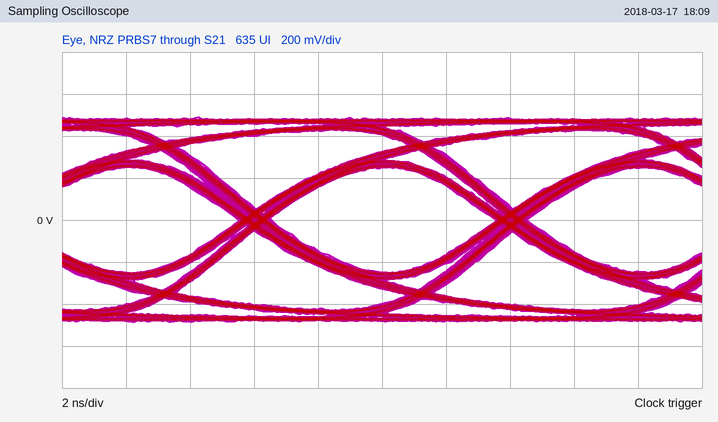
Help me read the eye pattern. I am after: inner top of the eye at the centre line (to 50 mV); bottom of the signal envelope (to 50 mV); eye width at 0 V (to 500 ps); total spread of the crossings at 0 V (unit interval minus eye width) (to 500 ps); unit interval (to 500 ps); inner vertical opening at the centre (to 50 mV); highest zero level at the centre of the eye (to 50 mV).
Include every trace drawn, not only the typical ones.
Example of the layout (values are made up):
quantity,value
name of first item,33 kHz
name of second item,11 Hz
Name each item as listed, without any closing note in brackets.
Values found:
quantity,value
inner top of the eye at the centre line,250 mV
bottom of the signal envelope,-500 mV
eye width at 0 V,7.0 ns
total spread of the crossings at 0 V (unit interval minus eye width),1.0 ns
unit interval,8.0 ns
inner vertical opening at the centre,500 mV
highest zero level at the centre of the eye,-250 mV
